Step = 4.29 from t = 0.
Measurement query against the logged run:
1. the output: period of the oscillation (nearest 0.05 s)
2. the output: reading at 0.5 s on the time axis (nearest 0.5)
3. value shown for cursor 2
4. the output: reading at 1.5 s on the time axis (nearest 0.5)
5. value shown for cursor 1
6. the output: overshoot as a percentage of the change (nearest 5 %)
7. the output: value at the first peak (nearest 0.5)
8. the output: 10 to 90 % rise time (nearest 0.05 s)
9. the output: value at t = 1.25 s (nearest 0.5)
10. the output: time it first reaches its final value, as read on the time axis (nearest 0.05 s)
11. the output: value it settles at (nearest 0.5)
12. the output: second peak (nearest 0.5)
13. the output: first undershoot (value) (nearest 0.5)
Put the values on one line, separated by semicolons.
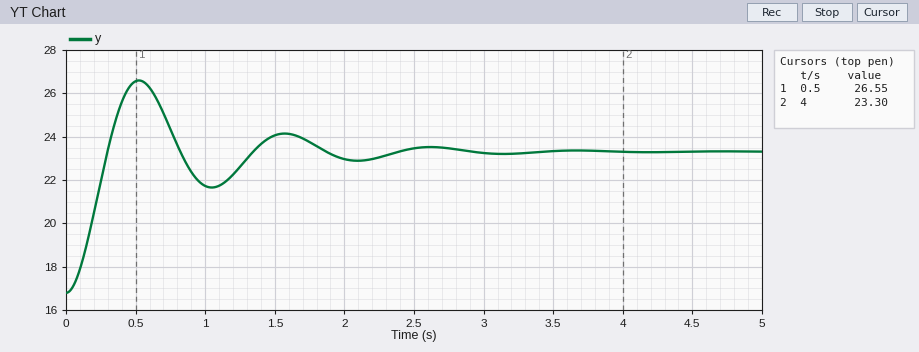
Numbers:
1.05 s; 26.5; 23.30; 24.0; 26.55; 50 %; 26.5; 0.20 s; 22.5; 0.30 s; 23.5; 24.0; 21.5
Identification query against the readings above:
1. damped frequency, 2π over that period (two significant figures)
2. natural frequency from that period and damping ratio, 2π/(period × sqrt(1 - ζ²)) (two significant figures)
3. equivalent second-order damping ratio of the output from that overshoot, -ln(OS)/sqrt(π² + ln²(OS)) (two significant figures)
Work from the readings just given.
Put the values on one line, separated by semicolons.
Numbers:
6.0 rad/s; 6.1 rad/s; 0.22
